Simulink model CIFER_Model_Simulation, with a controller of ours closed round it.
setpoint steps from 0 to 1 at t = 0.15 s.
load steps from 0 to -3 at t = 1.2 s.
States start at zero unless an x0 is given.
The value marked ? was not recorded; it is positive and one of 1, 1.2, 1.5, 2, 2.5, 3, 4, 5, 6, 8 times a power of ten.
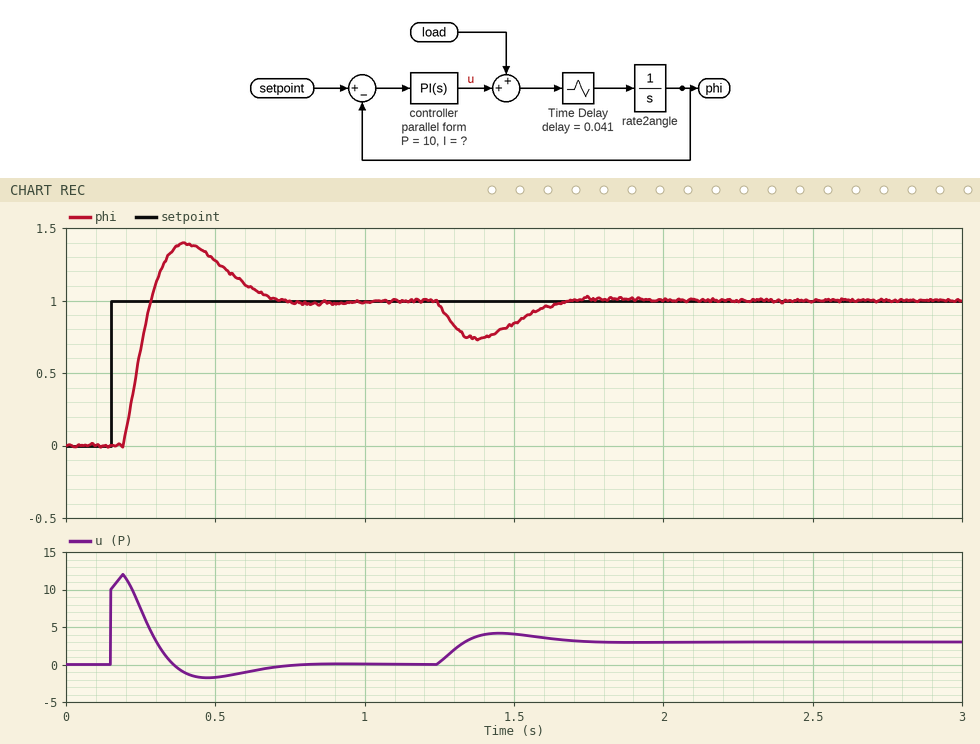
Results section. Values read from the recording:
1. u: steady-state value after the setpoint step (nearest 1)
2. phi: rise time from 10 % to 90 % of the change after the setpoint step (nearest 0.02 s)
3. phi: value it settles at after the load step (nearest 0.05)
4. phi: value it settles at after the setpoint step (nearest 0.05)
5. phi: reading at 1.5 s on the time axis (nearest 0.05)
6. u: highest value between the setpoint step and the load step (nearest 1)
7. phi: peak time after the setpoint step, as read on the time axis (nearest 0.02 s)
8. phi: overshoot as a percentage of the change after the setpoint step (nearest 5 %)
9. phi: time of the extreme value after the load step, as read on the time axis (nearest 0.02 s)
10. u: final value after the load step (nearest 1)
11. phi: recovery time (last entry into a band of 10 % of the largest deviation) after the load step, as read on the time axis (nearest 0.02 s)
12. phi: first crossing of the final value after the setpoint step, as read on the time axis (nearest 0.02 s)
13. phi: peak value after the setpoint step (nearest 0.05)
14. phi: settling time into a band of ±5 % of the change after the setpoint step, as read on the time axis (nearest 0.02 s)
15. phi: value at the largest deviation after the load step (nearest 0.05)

0
0.08 s
1.00
1.00
0.85
12
0.40 s
40 %
1.38 s
3
1.64 s
0.28 s
1.40
0.66 s
0.75
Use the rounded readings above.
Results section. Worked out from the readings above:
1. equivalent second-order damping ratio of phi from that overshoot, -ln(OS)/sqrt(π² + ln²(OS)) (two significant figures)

0.28
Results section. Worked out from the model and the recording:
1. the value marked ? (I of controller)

50
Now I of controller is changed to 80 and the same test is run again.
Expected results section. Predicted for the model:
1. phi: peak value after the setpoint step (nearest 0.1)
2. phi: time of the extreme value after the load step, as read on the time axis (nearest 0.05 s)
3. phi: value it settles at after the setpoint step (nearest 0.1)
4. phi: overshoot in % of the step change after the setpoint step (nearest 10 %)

1.6
1.35 s
1.0
60 %
